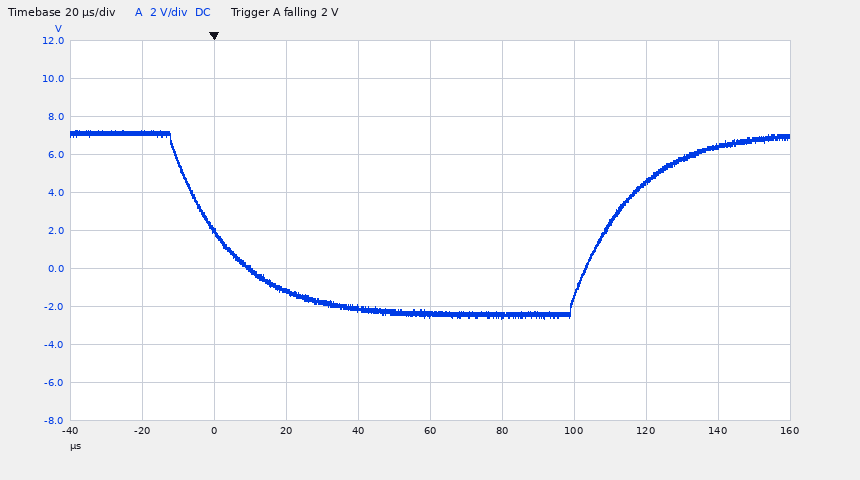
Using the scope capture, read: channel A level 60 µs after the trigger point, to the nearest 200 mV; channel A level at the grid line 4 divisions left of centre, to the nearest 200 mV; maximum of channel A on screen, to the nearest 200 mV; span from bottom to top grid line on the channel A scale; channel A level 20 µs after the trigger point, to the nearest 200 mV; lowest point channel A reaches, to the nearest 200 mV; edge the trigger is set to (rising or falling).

-2.4 V
7.2 V
7.2 V
20 V
-1.2 V
-2.6 V
falling
